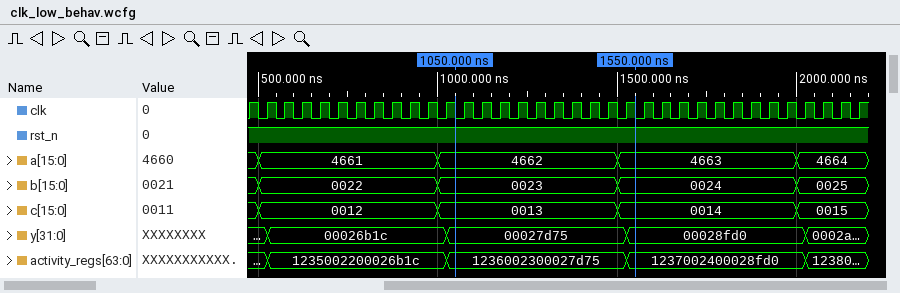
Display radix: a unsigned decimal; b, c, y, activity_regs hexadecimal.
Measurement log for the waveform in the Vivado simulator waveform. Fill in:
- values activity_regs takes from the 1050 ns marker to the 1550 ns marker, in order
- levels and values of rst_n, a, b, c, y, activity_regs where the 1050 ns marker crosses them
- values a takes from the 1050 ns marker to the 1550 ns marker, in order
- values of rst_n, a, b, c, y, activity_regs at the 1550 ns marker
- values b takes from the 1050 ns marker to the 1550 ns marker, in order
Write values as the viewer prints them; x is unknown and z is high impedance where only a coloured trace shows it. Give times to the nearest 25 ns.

1236002300027d75, 1237002400028fd0
rst_n=1, a=4662, b=0023, c=0013, y=00027d75, activity_regs=1236002300027d75
4662, 4663
rst_n=1, a=4663, b=0024, c=0014, y=00028fd0, activity_regs=1237002400028fd0
0023, 0024
